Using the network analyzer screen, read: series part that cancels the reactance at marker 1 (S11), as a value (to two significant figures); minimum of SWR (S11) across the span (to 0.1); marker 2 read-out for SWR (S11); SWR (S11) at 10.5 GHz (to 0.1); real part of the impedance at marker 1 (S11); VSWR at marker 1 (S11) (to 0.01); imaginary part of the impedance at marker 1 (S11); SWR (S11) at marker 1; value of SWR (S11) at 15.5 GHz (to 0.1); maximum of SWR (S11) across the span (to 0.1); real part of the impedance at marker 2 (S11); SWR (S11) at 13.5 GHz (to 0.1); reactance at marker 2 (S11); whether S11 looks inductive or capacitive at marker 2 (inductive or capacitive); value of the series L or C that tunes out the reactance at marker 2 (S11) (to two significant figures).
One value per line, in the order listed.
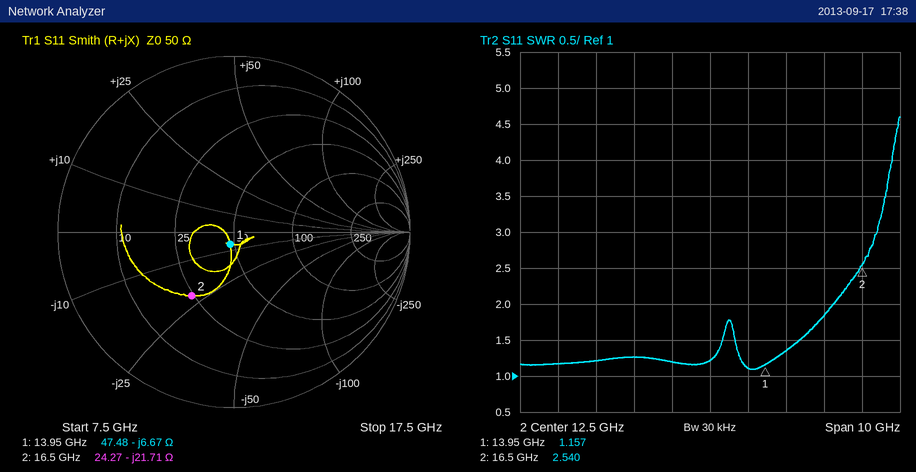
76 pH
1.1
2.540
1.3
47.48 Ω
1.16
-6.67 Ω
1.157
1.8
4.6
24.27 Ω
1.1
-21.71 Ω
capacitive
210 pH
